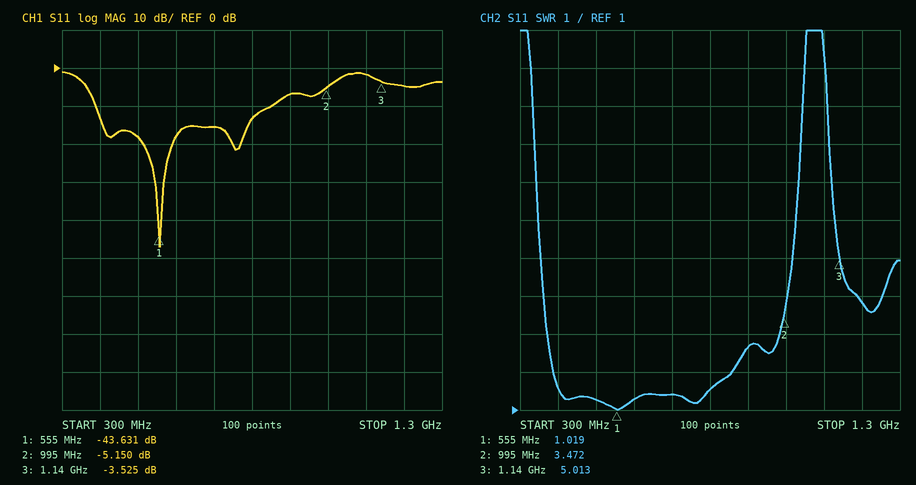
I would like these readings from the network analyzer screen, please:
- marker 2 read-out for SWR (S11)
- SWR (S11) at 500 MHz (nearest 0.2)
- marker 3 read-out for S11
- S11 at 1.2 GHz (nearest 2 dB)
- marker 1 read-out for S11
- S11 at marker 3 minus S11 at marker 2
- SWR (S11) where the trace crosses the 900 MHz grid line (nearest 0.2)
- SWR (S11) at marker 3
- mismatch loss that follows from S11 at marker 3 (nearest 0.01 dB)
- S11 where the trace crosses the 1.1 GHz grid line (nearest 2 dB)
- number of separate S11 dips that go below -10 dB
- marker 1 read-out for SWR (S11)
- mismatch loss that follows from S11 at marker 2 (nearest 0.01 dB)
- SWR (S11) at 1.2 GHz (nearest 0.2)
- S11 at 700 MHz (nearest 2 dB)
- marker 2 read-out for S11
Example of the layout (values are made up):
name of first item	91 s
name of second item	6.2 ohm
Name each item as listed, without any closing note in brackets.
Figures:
marker 2 read-out for SWR	3.472
SWR (S11) at 500 MHz	1.2
marker 3 read-out for S11	-3.525 dB
S11 at 1.2 GHz	-4 dB
marker 1 read-out for S11	-43.631 dB
S11 at marker 3 minus S11 at marker 2	1.625 dB
SWR (S11) where the trace crosses the 900 MHz grid line	2.6
SWR (S11) at marker 3	5.013
mismatch loss that follows from S11 at marker 3	2.55 dB
S11 where the trace crosses the 1.1 GHz grid line	-2 dB
number of separate S11 dips that go below -10 dB	2
marker 1 read-out for SWR	1.019
mismatch loss that follows from S11 at marker 2	1.58 dB
SWR (S11) at 1.2 GHz	3.8
S11 at 700 MHz	-16 dB
marker 2 read-out for S11	-5.150 dB
